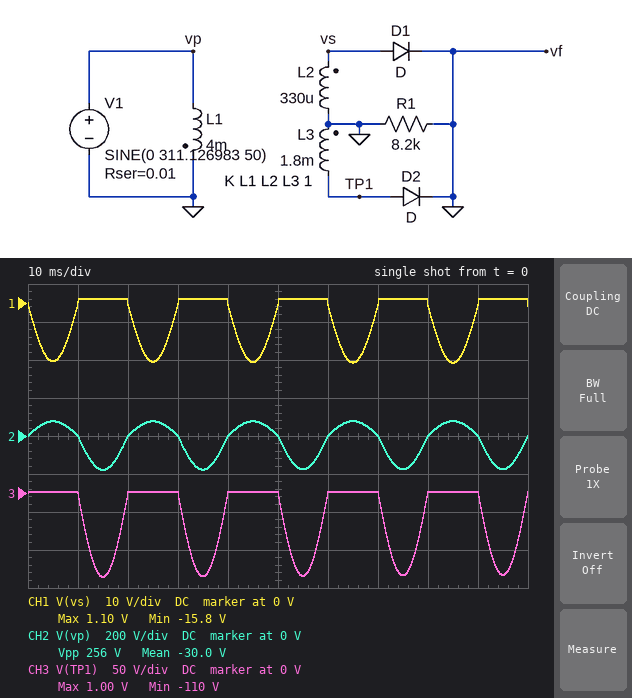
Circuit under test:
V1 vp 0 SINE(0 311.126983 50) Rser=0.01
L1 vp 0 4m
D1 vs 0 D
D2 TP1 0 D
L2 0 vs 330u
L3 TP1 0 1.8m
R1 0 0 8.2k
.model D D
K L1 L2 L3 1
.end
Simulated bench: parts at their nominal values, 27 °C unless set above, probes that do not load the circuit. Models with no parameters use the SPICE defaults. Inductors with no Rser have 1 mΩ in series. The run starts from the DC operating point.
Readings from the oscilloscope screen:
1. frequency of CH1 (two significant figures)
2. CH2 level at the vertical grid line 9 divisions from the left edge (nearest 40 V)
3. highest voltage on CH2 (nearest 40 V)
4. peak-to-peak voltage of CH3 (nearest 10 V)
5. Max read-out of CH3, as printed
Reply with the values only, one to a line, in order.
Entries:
50 Hz
0 V
80 V
110 V
1.00 V
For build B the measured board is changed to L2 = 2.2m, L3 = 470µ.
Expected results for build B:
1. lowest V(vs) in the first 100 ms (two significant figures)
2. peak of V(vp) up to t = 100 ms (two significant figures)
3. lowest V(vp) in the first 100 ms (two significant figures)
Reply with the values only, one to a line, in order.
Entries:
-100 V
150 V
-71 V
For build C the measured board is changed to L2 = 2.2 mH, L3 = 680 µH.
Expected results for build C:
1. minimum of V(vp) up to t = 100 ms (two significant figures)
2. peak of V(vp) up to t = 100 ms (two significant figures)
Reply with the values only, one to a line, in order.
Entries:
-70 V
130 V
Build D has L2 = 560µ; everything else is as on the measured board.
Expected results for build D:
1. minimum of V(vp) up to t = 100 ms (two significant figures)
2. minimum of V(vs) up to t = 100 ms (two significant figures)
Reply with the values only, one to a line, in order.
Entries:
-140 V
-20 V
